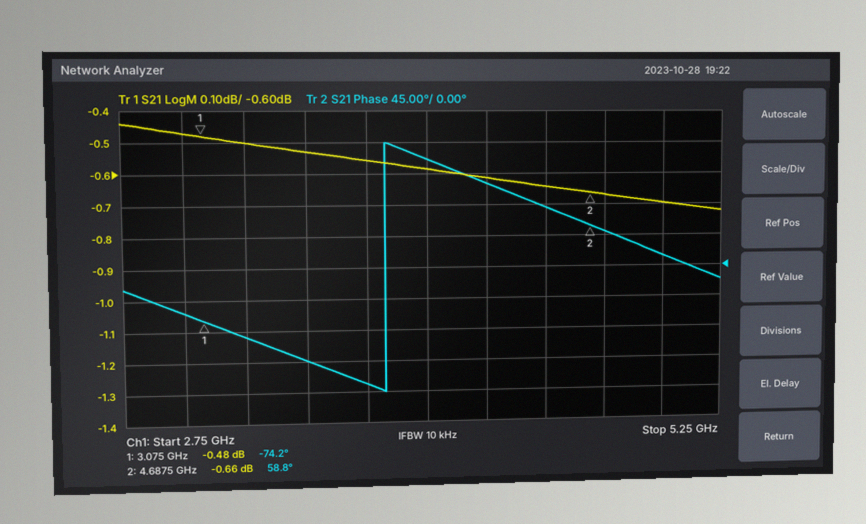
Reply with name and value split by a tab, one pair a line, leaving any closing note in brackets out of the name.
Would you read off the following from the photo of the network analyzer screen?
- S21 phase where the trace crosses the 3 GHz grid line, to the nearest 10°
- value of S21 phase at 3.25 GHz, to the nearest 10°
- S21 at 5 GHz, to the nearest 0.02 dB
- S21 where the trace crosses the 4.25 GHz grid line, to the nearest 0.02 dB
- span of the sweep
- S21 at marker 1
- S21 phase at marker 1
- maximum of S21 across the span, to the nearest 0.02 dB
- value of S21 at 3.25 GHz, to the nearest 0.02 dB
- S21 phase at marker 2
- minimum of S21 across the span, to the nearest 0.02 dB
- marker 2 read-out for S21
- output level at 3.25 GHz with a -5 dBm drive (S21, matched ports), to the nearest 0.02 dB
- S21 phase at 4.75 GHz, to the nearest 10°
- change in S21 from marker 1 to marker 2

S21 phase where the trace crosses the 3 GHz grid line, to the nearest 10°	-60°
value of S21 phase at 3.25 GHz, to the nearest 10°	-100°
S21 at 5 GHz, to the nearest 0.02 dB	-0.70 dB
S21 where the trace crosses the 4.25 GHz grid line, to the nearest 0.02 dB	-0.62 dB
span of the sweep	2.5 GHz
S21 at marker 1	-0.48 dB
S21 phase at marker 1	-74.2°
maximum of S21 across the span, to the nearest 0.02 dB	-0.44 dB
value of S21 at 3.25 GHz, to the nearest 0.02 dB	-0.50 dB
S21 phase at marker 2	58.8°
minimum of S21 across the span, to the nearest 0.02 dB	-0.72 dB
marker 2 read-out for S21	-0.66 dB
output level at 3.25 GHz with a -5 dBm drive (S21, matched ports), to the nearest 0.02 dB	-5.50 dBm
S21 phase at 4.75 GHz, to the nearest 10°	50°
change in S21 from marker 1 to marker 2	-0.18 dB
